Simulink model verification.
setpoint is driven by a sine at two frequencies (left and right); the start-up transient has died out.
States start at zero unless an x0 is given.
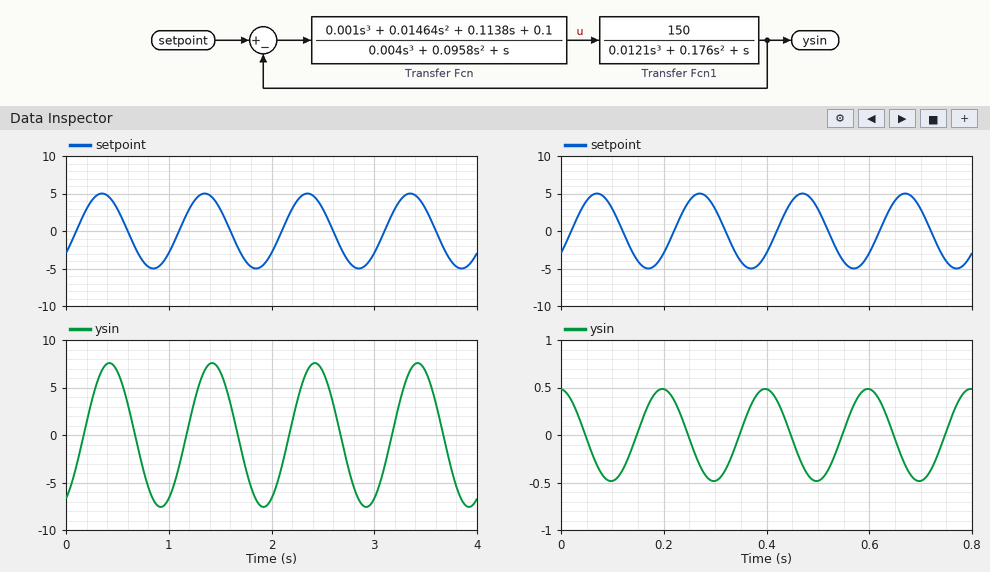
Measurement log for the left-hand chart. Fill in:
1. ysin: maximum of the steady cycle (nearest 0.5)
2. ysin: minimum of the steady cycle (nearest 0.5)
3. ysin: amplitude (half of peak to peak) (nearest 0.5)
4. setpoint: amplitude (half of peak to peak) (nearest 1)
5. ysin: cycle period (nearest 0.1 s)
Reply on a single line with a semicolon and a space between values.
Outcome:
7.5; -7.5; 7.5; 5; 1.0 s
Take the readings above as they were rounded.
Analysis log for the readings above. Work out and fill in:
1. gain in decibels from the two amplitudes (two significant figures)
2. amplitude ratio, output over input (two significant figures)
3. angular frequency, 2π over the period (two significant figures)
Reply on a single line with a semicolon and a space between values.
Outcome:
3.5 dB; 1.5; 6.3 rad/s
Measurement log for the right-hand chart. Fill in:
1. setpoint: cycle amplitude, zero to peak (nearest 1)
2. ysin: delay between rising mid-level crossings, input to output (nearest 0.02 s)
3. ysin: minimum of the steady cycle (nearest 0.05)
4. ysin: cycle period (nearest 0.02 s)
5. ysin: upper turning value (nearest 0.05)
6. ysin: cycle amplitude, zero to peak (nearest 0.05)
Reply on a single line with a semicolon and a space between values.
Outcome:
5; 0.12 s; -0.50; 0.20 s; 0.50; 0.50
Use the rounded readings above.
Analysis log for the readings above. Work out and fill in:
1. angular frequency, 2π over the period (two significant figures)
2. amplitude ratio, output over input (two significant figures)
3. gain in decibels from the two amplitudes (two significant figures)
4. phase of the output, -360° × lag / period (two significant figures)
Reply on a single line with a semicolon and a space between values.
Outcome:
31 rad/s; 0.10; -20 dB; -220°
